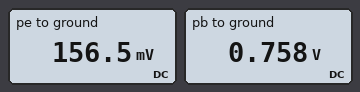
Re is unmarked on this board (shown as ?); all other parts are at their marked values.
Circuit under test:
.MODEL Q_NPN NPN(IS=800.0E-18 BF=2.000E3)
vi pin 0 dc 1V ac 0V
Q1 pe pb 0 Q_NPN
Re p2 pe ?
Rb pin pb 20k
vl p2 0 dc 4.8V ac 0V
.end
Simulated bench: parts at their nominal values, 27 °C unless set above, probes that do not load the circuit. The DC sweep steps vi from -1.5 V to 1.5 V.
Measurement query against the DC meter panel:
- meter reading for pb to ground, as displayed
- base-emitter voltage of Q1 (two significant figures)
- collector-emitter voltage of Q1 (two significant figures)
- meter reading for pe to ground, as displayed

0.758 V
760 mV
160 mV
156.5 mV
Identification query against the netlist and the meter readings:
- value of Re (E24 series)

1.1 kΩ
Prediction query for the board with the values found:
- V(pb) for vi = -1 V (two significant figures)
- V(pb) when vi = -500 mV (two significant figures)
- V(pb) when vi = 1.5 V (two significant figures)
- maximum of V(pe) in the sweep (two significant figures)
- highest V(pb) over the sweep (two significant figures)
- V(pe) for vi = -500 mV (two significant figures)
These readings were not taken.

-1.0 V
-500 mV
760 mV
4.8 V
760 mV
4.8 V
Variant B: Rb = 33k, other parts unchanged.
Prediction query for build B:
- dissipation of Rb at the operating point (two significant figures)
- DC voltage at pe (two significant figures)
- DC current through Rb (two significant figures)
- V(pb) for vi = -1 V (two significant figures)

1.8 µW
170 mV
7.3 µA
-1.0 V
